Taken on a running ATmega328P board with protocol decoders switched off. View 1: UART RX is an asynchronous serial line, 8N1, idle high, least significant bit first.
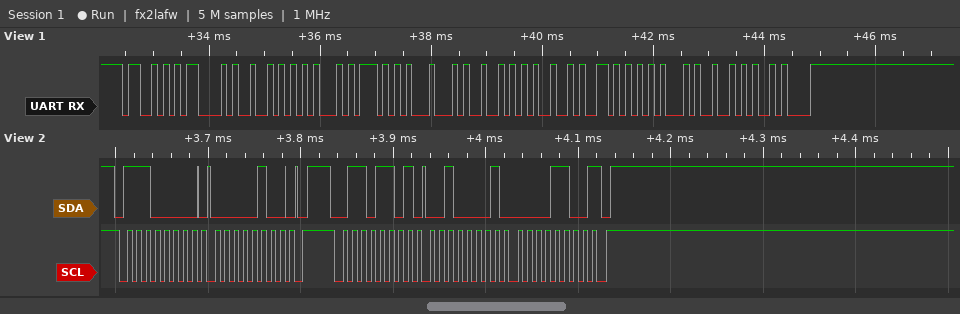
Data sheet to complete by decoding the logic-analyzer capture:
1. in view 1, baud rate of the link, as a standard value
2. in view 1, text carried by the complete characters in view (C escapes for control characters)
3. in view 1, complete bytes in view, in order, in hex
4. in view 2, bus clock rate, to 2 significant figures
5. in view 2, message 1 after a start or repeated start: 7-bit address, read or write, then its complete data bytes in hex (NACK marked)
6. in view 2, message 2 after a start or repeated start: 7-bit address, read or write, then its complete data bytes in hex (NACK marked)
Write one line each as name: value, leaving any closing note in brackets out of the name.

in view 1, baud rate of the link, as a standard value: 9600 baud
in view 1, text carried by the complete characters in view: "SCREWDRIVER\n"
in view 1, complete bytes in view, in order, in hex: 0x53 0x43 0x52 0x45 0x57 0x44 0x52 0x49 0x56 0x45 0x52 0x0A
in view 2, bus clock rate, to 2 significant figures: 100 kHz
in view 2, message 1 after a start or repeated start: 7-bit address, read or write, then its complete data bytes in hex: 0x70 write: 04
in view 2, message 2 after a start or repeated start: 7-bit address, read or write, then its complete data bytes in hex: 0x36 read: 21 0C NACK
